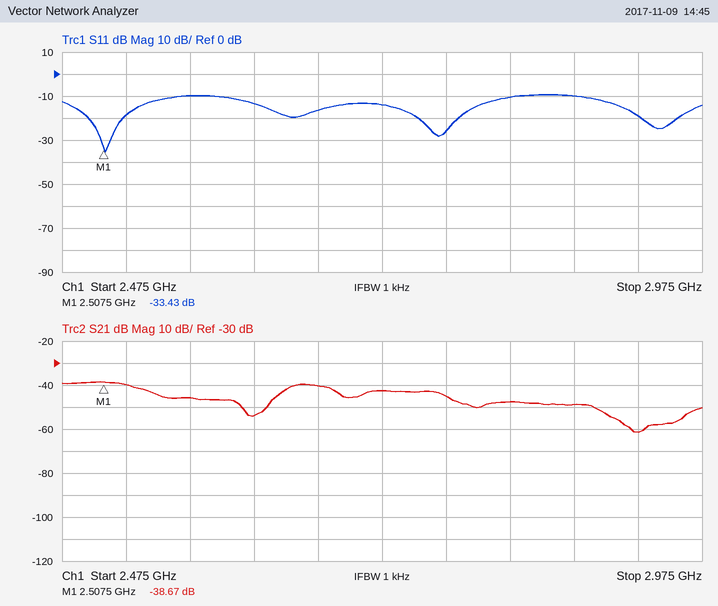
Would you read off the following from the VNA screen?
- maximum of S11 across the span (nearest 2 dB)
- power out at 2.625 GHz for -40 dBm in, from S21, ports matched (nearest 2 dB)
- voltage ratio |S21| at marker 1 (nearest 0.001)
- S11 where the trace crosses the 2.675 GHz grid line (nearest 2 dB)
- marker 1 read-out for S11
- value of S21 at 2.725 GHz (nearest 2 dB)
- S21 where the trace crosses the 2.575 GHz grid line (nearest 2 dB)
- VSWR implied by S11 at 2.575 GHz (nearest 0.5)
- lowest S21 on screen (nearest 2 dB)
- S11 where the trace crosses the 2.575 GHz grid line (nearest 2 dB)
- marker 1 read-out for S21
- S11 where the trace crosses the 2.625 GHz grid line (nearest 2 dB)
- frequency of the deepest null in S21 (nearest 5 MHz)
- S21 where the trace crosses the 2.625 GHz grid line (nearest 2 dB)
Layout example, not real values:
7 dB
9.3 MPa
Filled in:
-10 dB
-94 dBm
0.012
-16 dB
-33.43 dB
-42 dB
-46 dB
2.0
-62 dB
-10 dB
-38.67 dB
-14 dB
2.925 GHz
-54 dB
